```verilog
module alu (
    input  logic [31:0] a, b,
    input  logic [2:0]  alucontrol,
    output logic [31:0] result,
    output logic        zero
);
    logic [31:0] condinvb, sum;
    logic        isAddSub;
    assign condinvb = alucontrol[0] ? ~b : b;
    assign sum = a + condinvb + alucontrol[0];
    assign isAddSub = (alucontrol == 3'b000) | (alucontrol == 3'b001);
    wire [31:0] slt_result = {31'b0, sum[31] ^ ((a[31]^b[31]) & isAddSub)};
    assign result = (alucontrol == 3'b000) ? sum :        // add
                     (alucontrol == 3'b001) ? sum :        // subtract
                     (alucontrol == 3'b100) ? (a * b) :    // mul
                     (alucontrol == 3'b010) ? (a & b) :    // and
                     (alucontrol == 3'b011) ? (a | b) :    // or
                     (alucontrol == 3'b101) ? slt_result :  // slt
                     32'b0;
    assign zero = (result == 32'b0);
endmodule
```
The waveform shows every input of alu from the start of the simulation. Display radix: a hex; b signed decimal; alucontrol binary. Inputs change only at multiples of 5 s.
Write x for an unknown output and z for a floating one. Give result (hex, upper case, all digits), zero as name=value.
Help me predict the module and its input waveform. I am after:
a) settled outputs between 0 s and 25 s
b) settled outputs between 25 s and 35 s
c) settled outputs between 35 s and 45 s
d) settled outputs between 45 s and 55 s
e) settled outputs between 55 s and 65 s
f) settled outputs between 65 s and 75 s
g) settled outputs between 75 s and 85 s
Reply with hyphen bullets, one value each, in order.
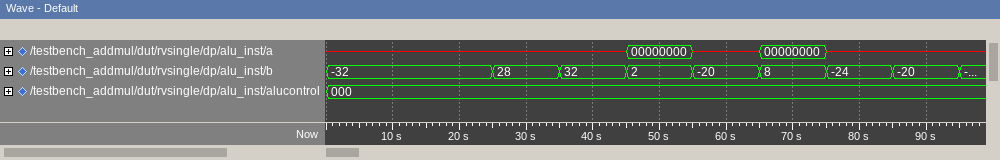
- result=x, zero=x
- result=x, zero=x
- result=x, zero=x
- result=00000002, zero=0
- result=x, zero=x
- result=00000008, zero=0
- result=x, zero=x
